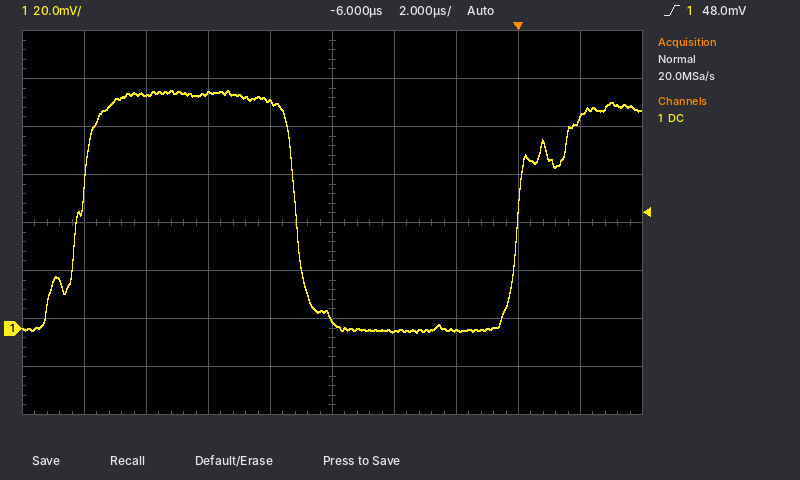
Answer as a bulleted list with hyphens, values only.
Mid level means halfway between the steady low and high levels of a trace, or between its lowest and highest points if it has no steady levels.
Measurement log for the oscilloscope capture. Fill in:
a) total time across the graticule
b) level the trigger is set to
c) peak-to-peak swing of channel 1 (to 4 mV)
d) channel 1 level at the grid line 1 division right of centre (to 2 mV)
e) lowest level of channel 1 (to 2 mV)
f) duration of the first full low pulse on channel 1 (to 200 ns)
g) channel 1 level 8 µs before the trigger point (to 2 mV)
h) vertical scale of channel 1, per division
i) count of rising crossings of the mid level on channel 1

- 20 µs
- 48.0 mV
- 100 mV
- -2 mV
- -2 mV
- 7.2 µs
- 94 mV
- 20 mV
- 2
